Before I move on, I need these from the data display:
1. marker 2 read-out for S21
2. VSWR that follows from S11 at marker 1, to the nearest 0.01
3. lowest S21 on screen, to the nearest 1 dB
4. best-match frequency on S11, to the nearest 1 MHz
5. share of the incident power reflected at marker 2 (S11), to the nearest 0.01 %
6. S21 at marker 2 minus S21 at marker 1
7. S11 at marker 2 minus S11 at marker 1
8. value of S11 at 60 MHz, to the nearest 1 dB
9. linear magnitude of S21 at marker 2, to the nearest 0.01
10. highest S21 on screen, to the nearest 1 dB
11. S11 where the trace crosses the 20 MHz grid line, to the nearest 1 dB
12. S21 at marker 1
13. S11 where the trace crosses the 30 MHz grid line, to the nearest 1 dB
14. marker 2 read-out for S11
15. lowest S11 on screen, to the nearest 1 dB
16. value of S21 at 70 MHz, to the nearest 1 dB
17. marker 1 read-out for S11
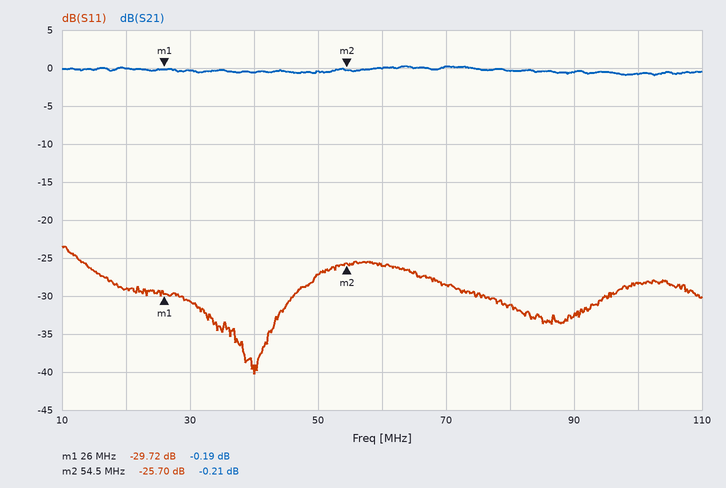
-0.21 dB
1.07
-1 dB
40 MHz
0.27 %
-0.02 dB
4.02 dB
-26 dB
0.98
0 dB
-29 dB
-0.19 dB
-31 dB
-25.70 dB
-40 dB
0 dB
-29.72 dB
